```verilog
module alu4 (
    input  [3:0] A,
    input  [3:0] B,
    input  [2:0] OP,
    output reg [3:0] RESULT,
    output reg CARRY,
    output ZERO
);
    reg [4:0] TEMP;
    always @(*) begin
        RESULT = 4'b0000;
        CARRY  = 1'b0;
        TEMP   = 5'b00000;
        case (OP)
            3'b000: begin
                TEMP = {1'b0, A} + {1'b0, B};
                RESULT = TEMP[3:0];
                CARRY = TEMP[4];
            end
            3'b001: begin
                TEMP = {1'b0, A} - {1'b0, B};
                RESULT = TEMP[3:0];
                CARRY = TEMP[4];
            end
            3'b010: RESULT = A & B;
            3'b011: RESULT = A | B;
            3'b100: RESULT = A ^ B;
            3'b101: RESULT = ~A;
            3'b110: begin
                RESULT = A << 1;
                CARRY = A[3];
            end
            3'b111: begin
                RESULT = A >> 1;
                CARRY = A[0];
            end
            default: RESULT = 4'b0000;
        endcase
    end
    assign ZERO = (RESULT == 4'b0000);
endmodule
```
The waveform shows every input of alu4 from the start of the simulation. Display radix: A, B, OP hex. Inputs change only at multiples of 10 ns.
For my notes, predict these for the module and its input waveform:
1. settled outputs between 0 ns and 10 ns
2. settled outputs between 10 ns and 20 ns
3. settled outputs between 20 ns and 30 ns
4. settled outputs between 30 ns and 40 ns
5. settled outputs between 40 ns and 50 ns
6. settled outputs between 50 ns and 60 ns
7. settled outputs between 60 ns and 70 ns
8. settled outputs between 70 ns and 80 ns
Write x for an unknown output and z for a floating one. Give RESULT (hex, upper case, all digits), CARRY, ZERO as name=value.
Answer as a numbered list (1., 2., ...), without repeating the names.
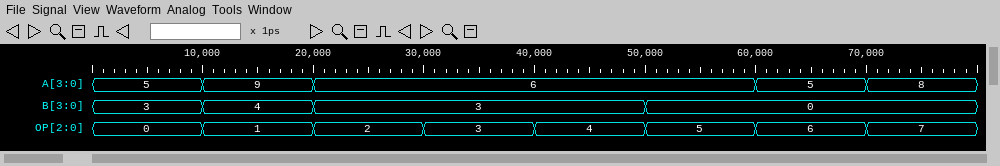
1. RESULT=8, CARRY=0, ZERO=0
2. RESULT=5, CARRY=0, ZERO=0
3. RESULT=2, CARRY=0, ZERO=0
4. RESULT=7, CARRY=0, ZERO=0
5. RESULT=5, CARRY=0, ZERO=0
6. RESULT=9, CARRY=0, ZERO=0
7. RESULT=A, CARRY=0, ZERO=0
8. RESULT=4, CARRY=0, ZERO=0
